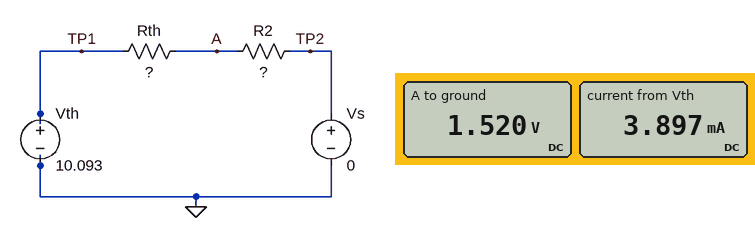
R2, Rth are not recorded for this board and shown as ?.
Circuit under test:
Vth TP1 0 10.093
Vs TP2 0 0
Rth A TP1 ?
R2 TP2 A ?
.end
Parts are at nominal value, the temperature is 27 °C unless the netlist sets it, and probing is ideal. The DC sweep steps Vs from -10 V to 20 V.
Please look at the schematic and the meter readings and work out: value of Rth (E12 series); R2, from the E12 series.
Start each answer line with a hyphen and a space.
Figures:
- 2.2 kΩ
- 390 Ω
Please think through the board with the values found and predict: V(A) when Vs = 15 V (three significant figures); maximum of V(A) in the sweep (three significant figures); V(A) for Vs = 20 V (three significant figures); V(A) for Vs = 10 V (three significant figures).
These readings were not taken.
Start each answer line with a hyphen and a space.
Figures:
- 14.3 V
- 18.5 V
- 18.5 V
- 10.0 V
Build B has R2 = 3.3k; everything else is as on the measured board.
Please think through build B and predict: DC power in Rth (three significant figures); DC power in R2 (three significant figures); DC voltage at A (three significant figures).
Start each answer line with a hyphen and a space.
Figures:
- 7.41 mW
- 11.1 mW
- 6.06 V
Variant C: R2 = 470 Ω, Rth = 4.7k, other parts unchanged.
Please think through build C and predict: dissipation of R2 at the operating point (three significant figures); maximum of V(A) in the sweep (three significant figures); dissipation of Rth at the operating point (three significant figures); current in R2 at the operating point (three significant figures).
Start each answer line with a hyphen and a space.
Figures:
- 1.79 mW
- 19.1 V
- 17.9 mW
- 1.95 mA
